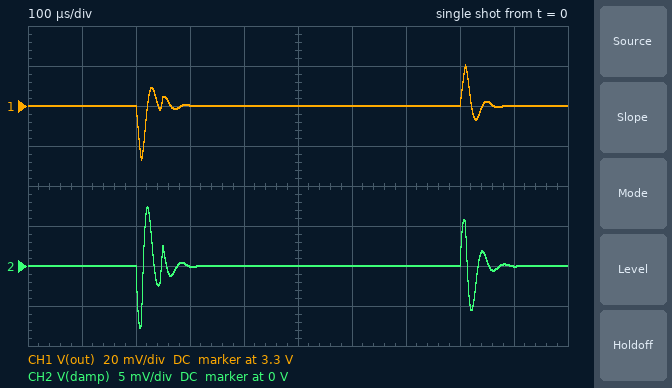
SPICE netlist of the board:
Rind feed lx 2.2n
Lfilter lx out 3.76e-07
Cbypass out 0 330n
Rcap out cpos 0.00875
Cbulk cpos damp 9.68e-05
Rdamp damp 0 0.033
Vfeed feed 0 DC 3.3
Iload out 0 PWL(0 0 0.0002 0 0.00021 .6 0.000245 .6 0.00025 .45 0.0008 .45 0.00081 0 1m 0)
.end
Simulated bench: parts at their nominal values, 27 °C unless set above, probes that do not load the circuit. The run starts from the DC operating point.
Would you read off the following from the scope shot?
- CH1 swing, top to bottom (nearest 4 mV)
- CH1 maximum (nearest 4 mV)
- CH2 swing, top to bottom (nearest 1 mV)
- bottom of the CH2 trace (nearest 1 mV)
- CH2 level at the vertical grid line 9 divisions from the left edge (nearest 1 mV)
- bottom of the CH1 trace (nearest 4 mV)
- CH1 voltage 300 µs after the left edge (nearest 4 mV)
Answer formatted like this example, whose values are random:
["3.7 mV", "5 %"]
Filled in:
["48 mV", "3.320 V", "15 mV", "-8 mV", "0 V", "3.272 V", "3.300 V"]
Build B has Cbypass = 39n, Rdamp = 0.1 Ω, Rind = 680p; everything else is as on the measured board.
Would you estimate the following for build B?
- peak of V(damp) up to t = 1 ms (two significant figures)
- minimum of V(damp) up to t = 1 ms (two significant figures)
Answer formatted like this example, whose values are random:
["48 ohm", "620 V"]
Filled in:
["11 mV", "-15 mV"]
